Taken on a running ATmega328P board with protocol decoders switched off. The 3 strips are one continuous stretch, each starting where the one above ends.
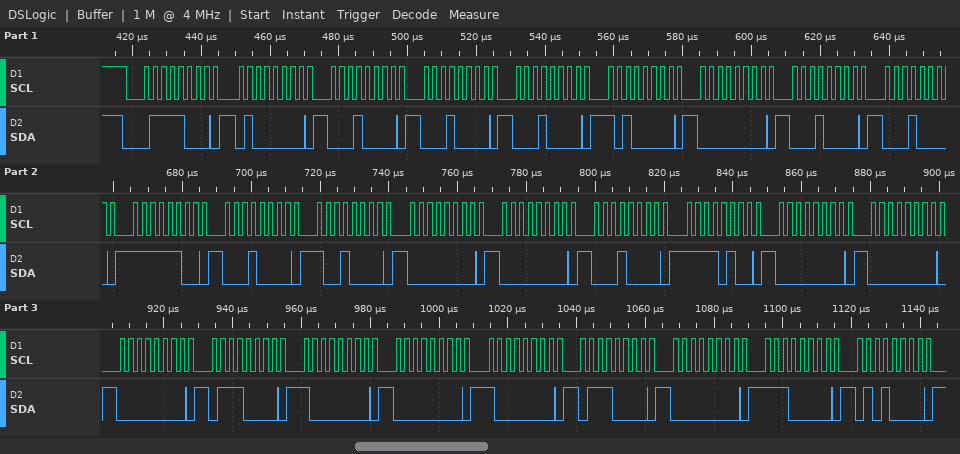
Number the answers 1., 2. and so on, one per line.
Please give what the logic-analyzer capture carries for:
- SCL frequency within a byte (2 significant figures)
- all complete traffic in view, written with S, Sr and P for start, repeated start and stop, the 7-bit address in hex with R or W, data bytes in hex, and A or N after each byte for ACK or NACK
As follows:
1. 400 kHz
2. S 3CW A 40 A 10 A 10 A 10 A A0 A 00 A 10 A 10 A FC A 10 A 90 A 00 A 00 A 10 A F4 A 00 A 00 A 00 A 70 A 80 A 00 A 80 A 70 A 00 A E0 A 50 A
